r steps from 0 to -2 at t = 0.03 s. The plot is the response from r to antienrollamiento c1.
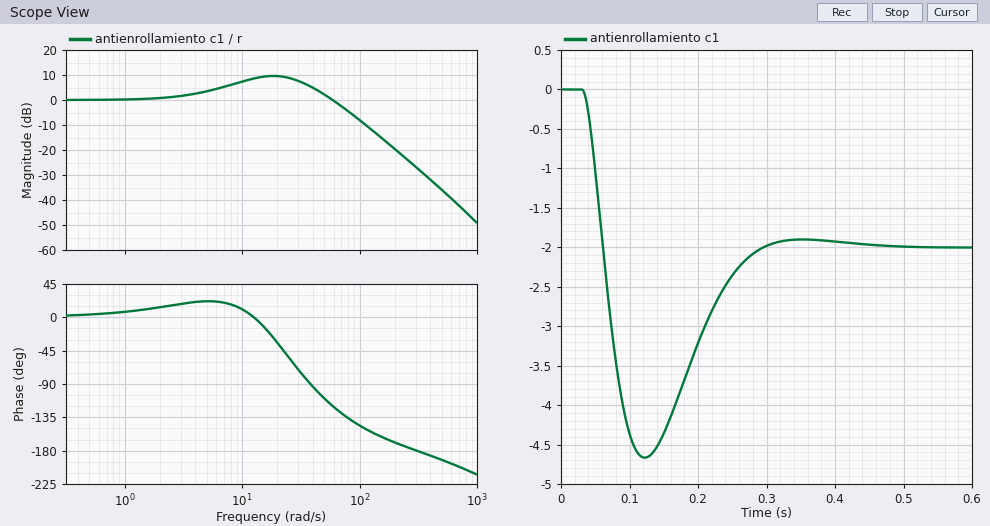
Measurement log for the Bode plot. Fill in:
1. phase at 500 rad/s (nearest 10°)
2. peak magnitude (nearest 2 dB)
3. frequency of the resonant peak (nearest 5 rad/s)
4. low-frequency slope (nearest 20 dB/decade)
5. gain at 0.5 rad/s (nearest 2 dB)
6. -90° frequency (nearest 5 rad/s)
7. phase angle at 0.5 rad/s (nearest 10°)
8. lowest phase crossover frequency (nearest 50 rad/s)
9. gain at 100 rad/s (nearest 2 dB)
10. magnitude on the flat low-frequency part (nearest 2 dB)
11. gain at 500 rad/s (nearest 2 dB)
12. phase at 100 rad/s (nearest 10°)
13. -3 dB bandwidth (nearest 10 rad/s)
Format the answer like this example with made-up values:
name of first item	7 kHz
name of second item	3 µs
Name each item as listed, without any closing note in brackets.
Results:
phase at 500 rad/s	-190°
peak magnitude	10 dB
frequency of the resonant peak	20 rad/s
low-frequency slope	0 dB/decade
gain at 0.5 rad/s	0 dB
-90° frequency	40 rad/s
phase angle at 0.5 rad/s	0°
lowest phase crossover frequency	300 rad/s
gain at 100 rad/s	-8 dB
magnitude on the flat low-frequency part	0 dB
gain at 500 rad/s	-36 dB
phase at 100 rad/s	-150°
-3 dB bandwidth	70 rad/s
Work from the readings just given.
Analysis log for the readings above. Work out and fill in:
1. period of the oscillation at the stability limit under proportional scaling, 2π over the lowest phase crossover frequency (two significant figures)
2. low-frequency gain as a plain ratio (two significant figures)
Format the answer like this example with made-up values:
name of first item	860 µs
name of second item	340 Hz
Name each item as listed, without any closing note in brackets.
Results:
period of the oscillation at the stability limit under proportional scaling, 2π over the lowest phase crossover frequency	0.021 s
low-frequency gain as a plain ratio	1.0
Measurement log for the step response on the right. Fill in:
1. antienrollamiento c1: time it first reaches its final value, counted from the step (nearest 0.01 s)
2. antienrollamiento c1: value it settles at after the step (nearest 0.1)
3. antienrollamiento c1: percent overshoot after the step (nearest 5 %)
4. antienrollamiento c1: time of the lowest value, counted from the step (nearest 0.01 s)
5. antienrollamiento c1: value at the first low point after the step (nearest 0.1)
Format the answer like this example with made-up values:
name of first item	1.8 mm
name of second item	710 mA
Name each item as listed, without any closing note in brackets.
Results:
antienrollamiento c1: time it first reaches its final value, counted from the step	0.03 s
antienrollamiento c1: value it settles at after the step	-2.0
antienrollamiento c1: percent overshoot after the step	135 %
antienrollamiento c1: time of the lowest value, counted from the step	0.09 s
antienrollamiento c1: value at the first low point after the step	-4.7
